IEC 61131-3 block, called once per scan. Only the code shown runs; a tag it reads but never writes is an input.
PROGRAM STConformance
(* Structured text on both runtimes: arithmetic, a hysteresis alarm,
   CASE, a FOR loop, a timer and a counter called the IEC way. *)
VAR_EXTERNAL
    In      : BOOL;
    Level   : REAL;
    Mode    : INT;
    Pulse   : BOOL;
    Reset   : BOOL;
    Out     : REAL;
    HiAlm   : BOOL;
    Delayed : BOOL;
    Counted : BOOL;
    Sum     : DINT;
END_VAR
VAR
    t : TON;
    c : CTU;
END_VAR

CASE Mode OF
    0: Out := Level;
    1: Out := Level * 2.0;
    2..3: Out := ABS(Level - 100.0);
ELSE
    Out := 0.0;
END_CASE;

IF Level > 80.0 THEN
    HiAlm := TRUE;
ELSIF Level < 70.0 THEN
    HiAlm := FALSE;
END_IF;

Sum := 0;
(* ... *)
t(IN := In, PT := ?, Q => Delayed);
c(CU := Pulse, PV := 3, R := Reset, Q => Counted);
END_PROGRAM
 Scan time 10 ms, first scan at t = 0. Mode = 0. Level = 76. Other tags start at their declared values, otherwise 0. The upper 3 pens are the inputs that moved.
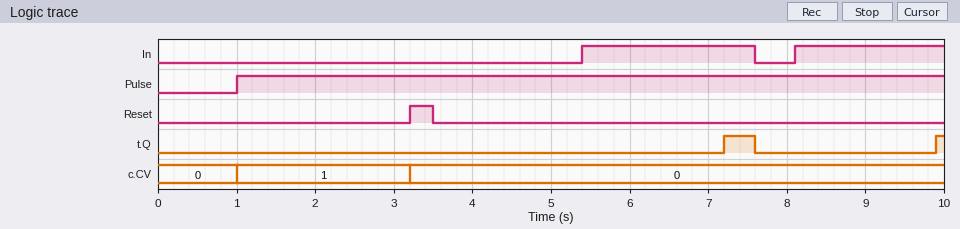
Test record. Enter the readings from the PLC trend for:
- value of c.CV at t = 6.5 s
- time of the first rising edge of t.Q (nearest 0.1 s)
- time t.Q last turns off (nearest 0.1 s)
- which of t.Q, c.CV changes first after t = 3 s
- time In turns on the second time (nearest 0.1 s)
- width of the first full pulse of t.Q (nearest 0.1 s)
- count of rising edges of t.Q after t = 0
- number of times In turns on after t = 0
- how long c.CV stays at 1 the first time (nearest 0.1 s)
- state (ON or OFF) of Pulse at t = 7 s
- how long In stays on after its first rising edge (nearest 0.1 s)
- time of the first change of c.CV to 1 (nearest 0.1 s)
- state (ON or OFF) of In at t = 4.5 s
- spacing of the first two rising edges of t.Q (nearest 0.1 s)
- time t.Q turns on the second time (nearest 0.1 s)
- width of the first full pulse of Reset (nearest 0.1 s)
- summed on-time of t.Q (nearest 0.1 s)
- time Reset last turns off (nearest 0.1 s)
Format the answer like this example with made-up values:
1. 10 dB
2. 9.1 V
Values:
1. 0
2. 7.2 s
3. 7.6 s
4. c.CV
5. 8.1 s
6. 0.4 s
7. 2
8. 2
9. 2.2 s
10. ON
11. 2.2 s
12. 1.0 s
13. OFF
14. 2.7 s
15. 9.9 s
16. 0.3 s
17. 0.5 s
18. 3.5 s
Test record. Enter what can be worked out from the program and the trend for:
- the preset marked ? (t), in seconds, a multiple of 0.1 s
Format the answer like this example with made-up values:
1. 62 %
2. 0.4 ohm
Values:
1. 1.8 s
